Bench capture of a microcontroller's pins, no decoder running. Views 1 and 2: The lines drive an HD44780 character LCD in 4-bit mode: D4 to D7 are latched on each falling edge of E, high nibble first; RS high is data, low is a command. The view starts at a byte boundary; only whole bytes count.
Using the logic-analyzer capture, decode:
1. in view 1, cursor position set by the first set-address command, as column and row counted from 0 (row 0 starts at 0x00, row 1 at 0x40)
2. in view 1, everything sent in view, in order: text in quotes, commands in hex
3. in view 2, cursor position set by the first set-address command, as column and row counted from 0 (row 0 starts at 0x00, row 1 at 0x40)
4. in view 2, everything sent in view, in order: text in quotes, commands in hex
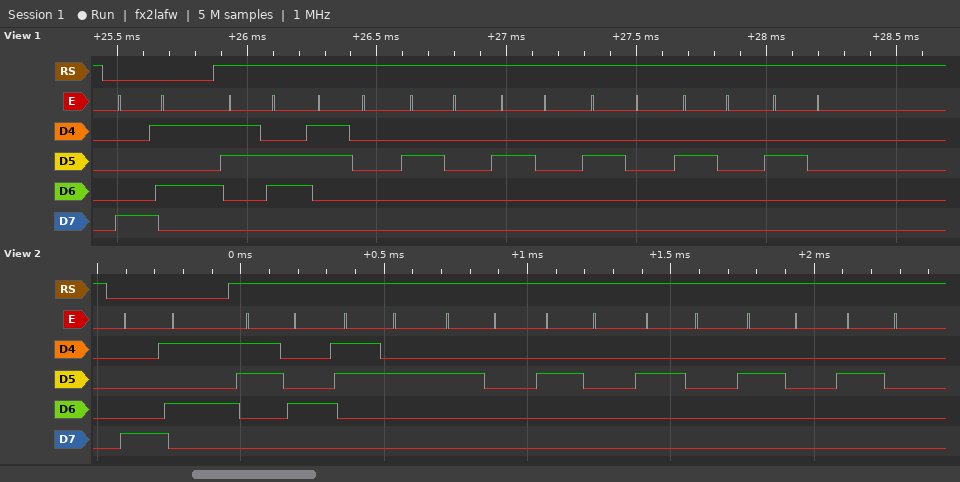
column 5, row 0
0x85 "60     "
column 5, row 0
0x85 "42     "
